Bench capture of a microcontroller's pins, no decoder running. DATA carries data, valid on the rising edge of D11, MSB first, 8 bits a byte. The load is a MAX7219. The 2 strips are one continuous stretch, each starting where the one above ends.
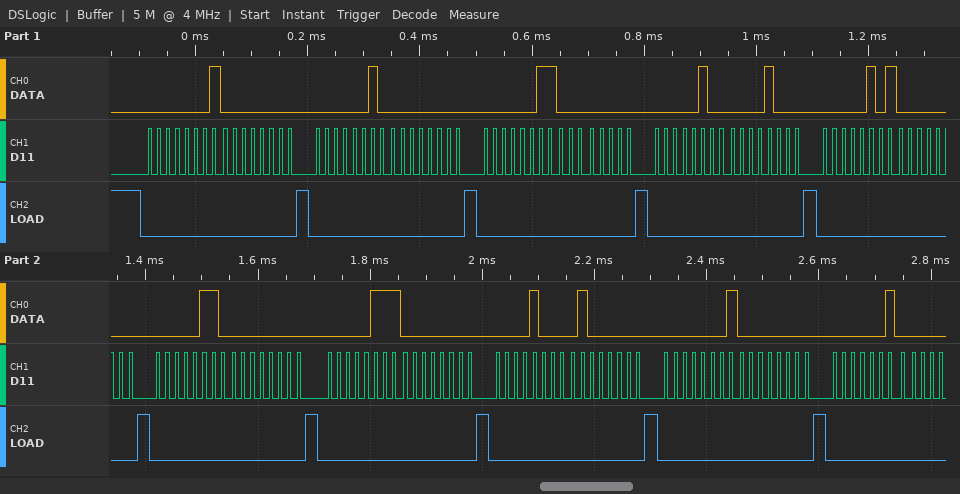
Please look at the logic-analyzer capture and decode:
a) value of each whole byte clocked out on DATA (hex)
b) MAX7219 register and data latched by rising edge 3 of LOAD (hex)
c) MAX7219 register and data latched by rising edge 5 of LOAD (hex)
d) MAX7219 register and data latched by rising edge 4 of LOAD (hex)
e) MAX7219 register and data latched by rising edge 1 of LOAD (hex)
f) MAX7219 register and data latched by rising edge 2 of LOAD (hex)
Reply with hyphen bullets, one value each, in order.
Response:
- 01 00 02 00 03 00 04 08 05 00 06 00 07 00 08 40 01 00 02
- register 0x3, data 0x00
- register 0x5, data 0x00
- register 0x4, data 0x08
- register 0x1, data 0x00
- register 0x2, data 0x00
